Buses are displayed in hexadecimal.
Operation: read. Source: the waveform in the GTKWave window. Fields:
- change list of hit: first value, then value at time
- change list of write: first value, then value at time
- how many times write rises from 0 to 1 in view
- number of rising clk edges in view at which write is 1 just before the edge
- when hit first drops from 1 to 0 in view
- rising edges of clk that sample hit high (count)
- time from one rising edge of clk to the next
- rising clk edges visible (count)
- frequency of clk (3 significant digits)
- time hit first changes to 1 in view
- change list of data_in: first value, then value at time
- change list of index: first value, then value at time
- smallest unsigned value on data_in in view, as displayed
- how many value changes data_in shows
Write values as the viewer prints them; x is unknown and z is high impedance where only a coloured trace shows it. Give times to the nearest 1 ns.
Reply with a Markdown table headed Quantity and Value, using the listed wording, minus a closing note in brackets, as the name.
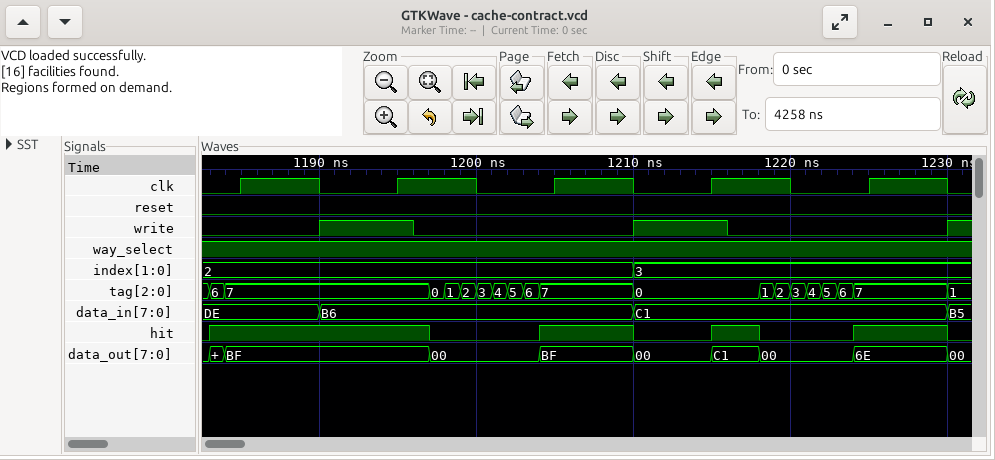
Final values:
| Quantity | Value |
|---|---|
| change list of hit: first value, then value at time | 0, 1 at 1183 ns, 0 at 1197 ns, 1 at 1204 ns, 0 at 1210 ns, 1 at 1215 ns, 0 at 1218 ns, 1 at 1224 ns, 0 at 1230 ns |
| change list of write: first value, then value at time | 0, 1 at 1190 ns, 0 at 1196 ns, 1 at 1210 ns, 0 at 1216 ns, 1 at 1230 ns |
| how many times write rises from 0 to 1 in view | 3 |
| number of rising clk edges in view at which write is 1 just before the edge | 2 |
| when hit first drops from 1 to 0 in view | 1197 ns |
| rising edges of clk that sample hit high | 4 |
| time from one rising edge of clk to the next | 10 ns |
| rising clk edges visible | 5 |
| frequency of clk | 100 MHz |
| time hit first changes to 1 in view | 1183 ns |
| change list of data_in: first value, then value at time | DE, B6 at 1190 ns, C1 at 1210 ns, B5 at 1230 ns |
| change list of index: first value, then value at time | 2, 3 at 1210 ns |
| smallest unsigned value on data_in in view, as displayed | B5 |
| how many value changes data_in shows | 3 |
